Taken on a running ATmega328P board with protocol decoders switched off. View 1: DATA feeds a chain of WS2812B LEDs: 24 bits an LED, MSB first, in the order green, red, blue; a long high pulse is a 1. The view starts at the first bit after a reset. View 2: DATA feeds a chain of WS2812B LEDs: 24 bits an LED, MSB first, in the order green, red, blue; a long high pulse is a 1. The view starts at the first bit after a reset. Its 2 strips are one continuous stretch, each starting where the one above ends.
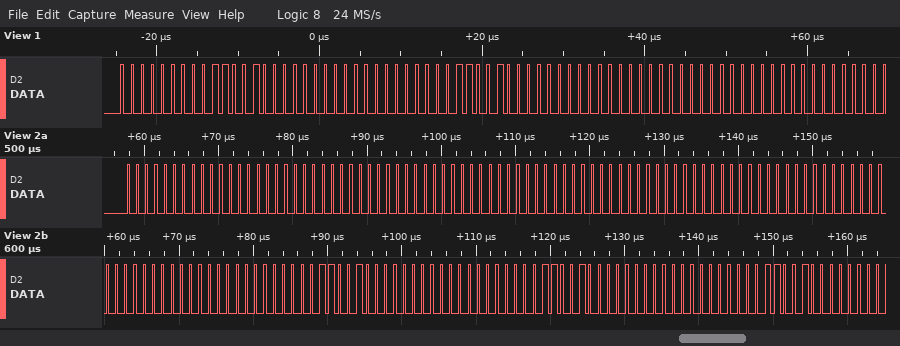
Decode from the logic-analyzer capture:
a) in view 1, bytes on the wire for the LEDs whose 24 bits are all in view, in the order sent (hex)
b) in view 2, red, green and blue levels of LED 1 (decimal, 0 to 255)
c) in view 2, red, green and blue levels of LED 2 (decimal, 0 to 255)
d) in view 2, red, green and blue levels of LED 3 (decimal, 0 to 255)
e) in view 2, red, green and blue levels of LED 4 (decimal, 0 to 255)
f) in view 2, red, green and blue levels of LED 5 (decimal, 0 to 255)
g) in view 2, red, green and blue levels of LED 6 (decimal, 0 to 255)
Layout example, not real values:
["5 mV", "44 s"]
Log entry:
["00 64 00 00 64 00 00 00 00", "0, 0, 0", "0, 0, 0", "0, 0, 0", "0, 0, 0", "100, 0, 0", "100, 0, 0"]
